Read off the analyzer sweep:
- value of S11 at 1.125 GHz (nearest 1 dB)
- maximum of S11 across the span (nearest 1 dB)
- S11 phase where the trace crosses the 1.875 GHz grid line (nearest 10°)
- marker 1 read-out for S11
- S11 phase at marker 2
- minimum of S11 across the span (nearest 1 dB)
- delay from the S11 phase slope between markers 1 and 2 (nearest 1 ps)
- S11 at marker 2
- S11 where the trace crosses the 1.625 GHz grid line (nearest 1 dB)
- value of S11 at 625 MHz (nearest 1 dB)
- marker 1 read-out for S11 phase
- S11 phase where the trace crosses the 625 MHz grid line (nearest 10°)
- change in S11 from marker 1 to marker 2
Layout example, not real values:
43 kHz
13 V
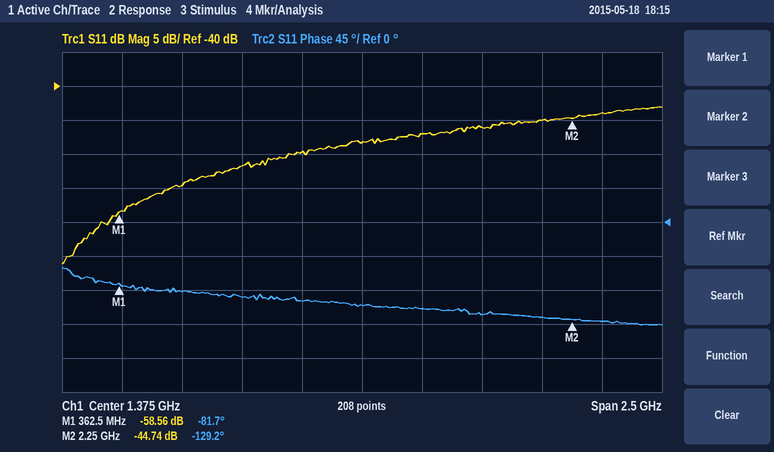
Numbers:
-50 dB
-43 dB
-120°
-58.56 dB
-129.2°
-66 dB
70 ps
-44.74 dB
-47 dB
-55 dB
-81.7°
-90°
13.82 dB
